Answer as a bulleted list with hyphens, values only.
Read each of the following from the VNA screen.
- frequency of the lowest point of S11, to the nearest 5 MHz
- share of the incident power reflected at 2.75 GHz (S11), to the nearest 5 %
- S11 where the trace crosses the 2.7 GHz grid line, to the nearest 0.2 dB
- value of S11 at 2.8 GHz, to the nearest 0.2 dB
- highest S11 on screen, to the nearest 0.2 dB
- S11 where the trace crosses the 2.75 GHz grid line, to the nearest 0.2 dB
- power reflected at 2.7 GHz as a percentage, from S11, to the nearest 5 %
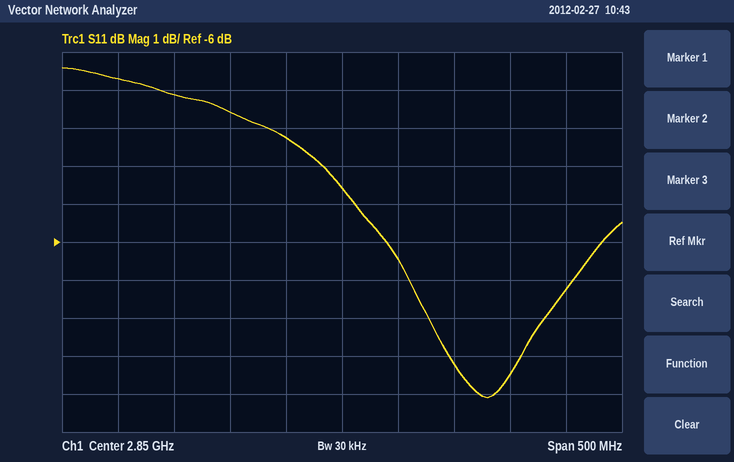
- 2.980 GHz
- 55 %
- -2.2 dB
- -3.2 dB
- -1.4 dB
- -2.6 dB
- 60 %
